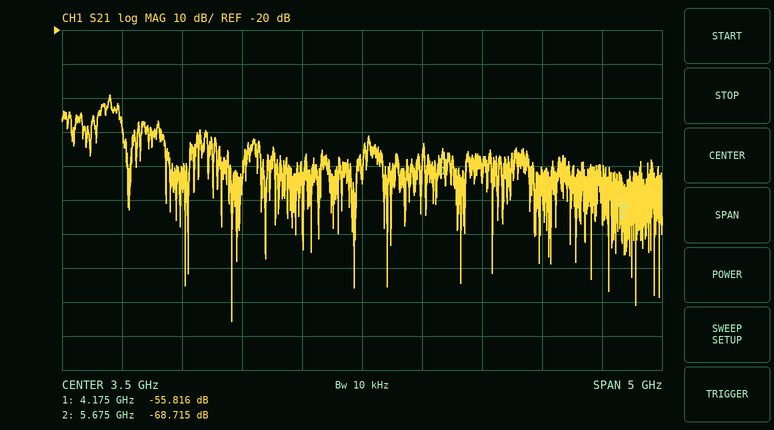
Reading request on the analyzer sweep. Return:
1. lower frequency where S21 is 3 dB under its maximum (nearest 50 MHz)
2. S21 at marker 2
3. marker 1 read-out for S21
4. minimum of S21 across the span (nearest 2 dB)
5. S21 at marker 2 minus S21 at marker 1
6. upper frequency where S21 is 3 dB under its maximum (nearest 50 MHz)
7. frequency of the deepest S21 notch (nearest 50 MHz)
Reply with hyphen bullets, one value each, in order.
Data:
- 1.40 GHz
- -68.715 dB
- -55.816 dB
- -106 dB
- -12.899 dB
- 1.40 GHz
- 2.40 GHz
